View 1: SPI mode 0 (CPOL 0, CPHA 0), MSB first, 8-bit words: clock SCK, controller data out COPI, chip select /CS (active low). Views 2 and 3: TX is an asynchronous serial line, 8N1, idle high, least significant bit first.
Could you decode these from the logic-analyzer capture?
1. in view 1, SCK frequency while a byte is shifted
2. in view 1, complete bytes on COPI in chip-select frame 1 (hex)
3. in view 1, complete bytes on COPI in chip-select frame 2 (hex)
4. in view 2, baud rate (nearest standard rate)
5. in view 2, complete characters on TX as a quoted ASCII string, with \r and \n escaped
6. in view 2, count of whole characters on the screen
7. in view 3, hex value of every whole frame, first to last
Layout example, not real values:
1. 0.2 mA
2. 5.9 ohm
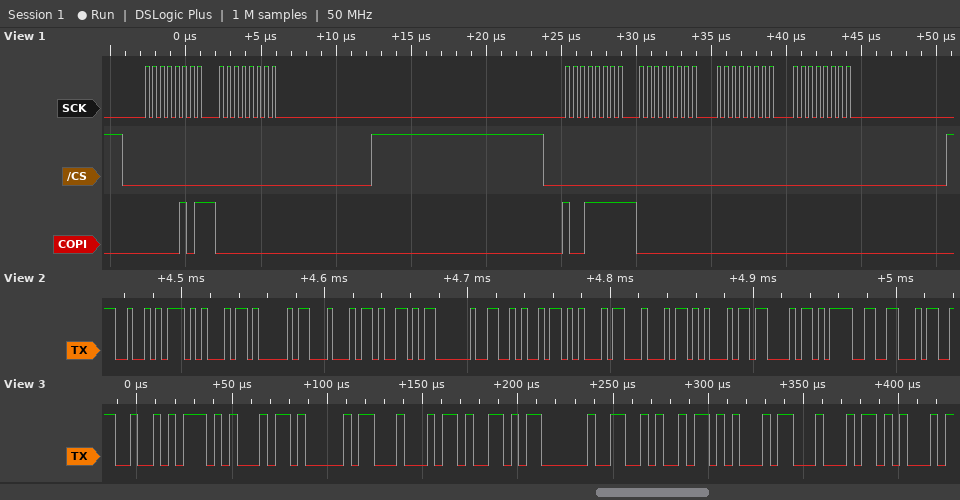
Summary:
1. 2 MHz
2. 0x05 0x00
3. 0x9F 0x00 0x00 0x00
4. 250000 baud
5. "READY JEDEC=F"
6. 13
7. 52 45 41 44 59 20 4A 45 44 45
